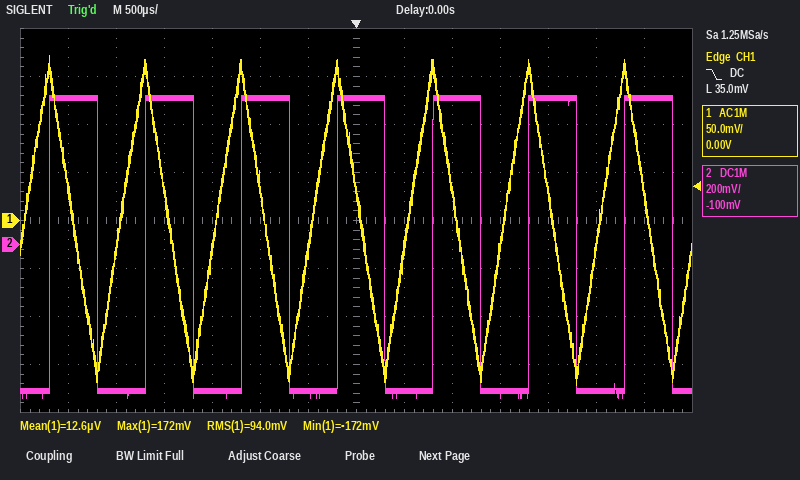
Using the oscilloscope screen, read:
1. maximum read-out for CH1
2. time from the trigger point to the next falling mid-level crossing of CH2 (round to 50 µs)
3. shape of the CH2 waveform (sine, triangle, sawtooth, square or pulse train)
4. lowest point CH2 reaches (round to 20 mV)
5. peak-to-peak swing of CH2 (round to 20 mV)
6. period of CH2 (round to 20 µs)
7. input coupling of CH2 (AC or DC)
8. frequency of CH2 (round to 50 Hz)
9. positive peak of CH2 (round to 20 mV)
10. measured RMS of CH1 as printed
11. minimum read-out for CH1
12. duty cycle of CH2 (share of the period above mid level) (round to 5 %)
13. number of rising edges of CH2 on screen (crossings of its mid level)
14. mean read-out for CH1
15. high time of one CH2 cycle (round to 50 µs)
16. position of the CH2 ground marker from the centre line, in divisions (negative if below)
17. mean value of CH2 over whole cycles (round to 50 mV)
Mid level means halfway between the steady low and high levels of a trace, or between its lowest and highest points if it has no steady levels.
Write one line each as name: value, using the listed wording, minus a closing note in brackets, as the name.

maximum read-out for CH1: 172 mV
time from the trigger point to the next falling mid-level crossing of CH2: 300 µs
shape of the CH2 waveform: square
lowest point CH2 reaches: -640 mV
peak-to-peak swing of CH2: 1.26 V
period of CH2: 1.00 ms
input coupling of CH2: DC
frequency of CH2: 1.00 kHz
positive peak of CH2: 620 mV
measured RMS of CH1 as printed: 94.0 mV
minimum read-out for CH1: -172 mV
duty cycle of CH2 (share of the period above mid level): 50 %
number of rising edges of CH2 on screen: 7
mean read-out for CH1: 12.6 µV
high time of one CH2 cycle: 500 µs
position of the CH2 ground marker from the centre line, in divisions: -0.5 div
mean value of CH2 over whole cycles: 0 mV
